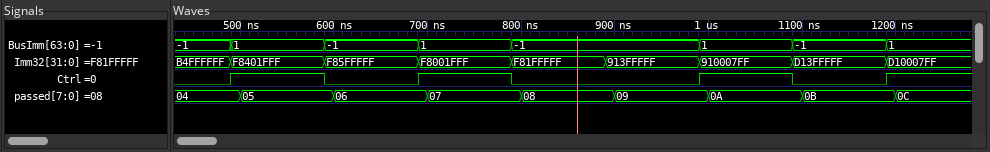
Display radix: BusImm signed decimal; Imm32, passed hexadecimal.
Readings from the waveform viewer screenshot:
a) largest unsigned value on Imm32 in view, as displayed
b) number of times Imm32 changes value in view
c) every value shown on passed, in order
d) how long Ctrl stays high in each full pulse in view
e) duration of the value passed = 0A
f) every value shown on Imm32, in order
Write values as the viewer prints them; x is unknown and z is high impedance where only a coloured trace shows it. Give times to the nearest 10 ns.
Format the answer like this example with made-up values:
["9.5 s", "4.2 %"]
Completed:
["F85FFFFF", "8", "04, 05, 06, 07, 08, 09, 0A, 0B, 0C", "100 ns, 100 ns, 100 ns", "100 ns", "B4FFFFFF, F8401FFF, F85FFFFF, F8001FFF, F81FFFFF, 913FFFFF, 910007FF, D13FFFFF, D10007FF"]
